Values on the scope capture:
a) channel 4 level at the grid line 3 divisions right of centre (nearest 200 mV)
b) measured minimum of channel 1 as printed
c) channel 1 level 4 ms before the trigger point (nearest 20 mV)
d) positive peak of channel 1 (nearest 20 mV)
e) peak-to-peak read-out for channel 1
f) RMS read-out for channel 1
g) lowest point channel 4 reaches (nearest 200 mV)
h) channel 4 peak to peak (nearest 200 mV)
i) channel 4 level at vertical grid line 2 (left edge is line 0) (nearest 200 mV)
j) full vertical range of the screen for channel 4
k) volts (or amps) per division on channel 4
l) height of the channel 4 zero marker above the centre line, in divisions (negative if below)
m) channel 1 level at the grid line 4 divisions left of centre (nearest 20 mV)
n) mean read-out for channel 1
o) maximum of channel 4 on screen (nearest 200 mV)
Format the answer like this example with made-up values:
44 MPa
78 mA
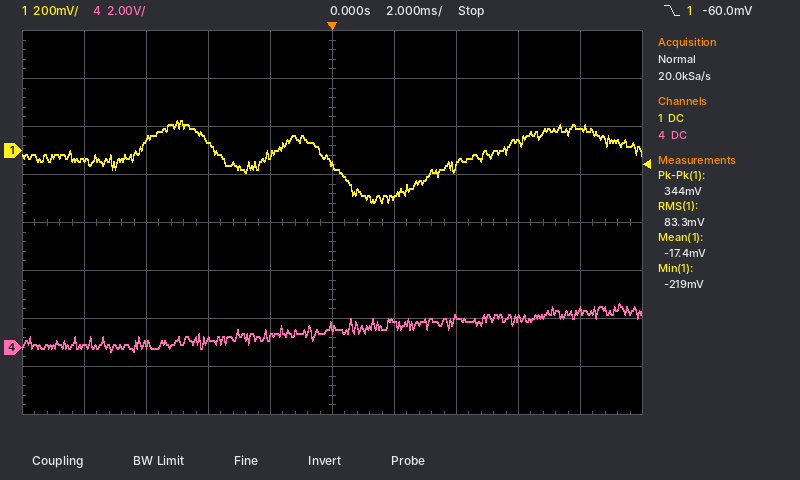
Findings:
1.2 V
-219 mV
40 mV
120 mV
344 mV
83.3 mV
-200 mV
2.0 V
200 mV
16 V
2 V
-2.6 div
-40 mV
-17.4 mV
1.8 V
